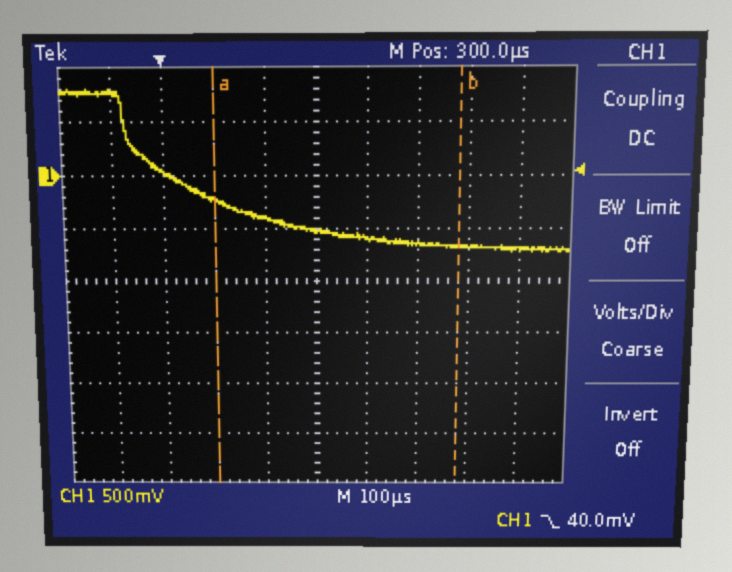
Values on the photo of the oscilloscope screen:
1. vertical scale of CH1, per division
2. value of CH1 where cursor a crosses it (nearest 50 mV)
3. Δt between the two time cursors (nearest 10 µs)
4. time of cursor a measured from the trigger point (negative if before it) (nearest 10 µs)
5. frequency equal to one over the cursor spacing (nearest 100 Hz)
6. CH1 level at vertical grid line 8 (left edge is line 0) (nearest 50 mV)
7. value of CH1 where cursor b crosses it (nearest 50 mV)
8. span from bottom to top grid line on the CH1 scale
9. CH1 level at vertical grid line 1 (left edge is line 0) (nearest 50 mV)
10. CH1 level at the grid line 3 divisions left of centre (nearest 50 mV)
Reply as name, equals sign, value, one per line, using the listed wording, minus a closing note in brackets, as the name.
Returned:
vertical scale of CH1, per division = 500 mV
value of CH1 where cursor a crosses it = -250 mV
Δt between the two time cursors = 480 µs
time of cursor a measured from the trigger point (negative if before it) = +100 µs
frequency equal to one over the cursor spacing = 2.1 kHz
CH1 level at vertical grid line 8 (left edge is line 0) = -650 mV
value of CH1 where cursor b crosses it = -650 mV
span from bottom to top grid line on the CH1 scale = 4 V
CH1 level at vertical grid line 1 (left edge is line 0) = 750 mV
CH1 level at the grid line 3 divisions left of centre = 50 mV
